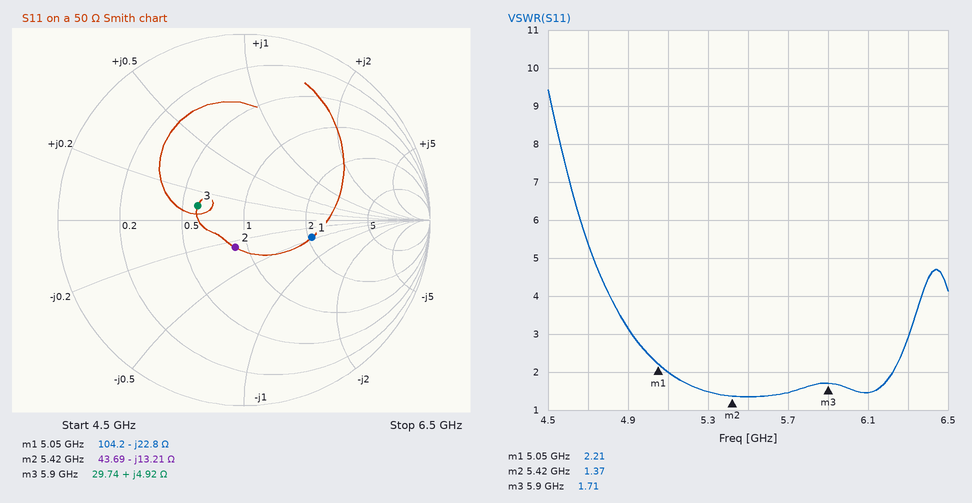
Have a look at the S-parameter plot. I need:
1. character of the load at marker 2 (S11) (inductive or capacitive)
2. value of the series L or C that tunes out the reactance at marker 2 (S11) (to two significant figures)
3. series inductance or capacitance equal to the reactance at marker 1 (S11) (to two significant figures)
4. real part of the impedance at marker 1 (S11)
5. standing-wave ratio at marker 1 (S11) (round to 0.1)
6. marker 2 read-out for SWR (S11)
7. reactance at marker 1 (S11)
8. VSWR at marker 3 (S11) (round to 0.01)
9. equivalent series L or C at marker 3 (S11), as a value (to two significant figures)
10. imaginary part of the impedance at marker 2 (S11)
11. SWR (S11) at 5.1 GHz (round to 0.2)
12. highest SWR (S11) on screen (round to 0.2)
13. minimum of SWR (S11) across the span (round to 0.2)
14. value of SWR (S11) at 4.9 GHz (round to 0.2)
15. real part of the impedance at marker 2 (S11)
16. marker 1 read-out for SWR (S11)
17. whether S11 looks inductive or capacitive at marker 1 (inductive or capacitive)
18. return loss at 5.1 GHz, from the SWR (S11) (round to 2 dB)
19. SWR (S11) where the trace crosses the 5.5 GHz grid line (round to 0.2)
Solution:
capacitive
390 pH
1.4 pF
104.2 Ω
2.2
1.37
-22.8 Ω
1.71
130 pH
-13.21 Ω
2.0
9.4
1.4
3.2
43.69 Ω
2.21
capacitive
10 dB
1.4
